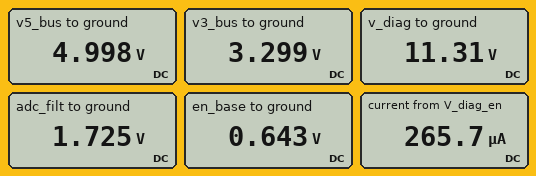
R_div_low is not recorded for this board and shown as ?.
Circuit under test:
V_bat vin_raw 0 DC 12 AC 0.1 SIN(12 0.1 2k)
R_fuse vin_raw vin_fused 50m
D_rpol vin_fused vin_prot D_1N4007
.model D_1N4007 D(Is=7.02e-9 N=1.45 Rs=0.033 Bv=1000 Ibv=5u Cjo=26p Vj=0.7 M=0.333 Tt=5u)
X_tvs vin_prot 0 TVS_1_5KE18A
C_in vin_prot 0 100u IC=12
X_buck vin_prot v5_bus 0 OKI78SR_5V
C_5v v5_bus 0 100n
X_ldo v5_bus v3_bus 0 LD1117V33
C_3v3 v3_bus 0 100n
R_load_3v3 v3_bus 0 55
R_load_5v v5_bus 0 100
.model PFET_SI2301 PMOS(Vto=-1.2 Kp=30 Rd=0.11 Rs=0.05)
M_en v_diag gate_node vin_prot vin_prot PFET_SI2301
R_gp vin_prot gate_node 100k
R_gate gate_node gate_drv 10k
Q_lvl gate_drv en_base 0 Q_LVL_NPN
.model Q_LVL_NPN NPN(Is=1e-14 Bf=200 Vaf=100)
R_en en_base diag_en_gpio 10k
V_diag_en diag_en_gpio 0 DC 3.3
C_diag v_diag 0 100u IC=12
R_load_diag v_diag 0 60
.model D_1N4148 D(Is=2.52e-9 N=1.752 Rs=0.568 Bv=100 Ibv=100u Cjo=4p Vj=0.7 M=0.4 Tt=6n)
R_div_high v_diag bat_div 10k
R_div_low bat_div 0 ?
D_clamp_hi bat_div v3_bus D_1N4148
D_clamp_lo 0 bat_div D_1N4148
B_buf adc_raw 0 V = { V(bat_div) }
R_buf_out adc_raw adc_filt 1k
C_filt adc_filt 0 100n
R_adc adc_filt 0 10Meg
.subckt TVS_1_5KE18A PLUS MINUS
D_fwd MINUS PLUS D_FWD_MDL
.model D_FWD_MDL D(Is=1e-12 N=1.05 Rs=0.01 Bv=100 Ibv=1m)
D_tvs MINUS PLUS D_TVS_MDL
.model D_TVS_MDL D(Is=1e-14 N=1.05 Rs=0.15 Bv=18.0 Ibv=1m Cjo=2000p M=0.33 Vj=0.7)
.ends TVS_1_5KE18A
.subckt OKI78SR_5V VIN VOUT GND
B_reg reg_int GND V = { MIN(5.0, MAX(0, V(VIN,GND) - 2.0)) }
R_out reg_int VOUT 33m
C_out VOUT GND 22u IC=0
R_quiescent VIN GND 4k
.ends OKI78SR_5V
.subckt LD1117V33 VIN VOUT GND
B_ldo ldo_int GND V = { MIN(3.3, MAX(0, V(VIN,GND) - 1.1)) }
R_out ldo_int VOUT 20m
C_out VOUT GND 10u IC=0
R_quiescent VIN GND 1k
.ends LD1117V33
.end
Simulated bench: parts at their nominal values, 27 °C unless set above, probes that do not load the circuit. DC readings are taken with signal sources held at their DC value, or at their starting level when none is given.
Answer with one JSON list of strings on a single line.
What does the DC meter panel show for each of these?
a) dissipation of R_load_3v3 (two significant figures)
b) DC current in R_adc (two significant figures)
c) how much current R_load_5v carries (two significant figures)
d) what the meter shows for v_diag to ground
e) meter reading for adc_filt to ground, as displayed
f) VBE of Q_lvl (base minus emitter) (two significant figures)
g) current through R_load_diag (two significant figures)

["200 mW", "170 nA", "50 mA", "11.31 V", "1.725 V", "640 mV", "190 mA"]
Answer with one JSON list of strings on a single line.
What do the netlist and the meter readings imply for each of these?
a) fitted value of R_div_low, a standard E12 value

["1.8 kΩ"]
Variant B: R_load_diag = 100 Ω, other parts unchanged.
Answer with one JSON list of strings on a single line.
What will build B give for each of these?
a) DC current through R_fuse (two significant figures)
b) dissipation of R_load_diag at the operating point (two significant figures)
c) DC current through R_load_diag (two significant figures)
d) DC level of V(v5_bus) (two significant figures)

["120 mA", "1.3 W", "110 mA", "5.0 V"]
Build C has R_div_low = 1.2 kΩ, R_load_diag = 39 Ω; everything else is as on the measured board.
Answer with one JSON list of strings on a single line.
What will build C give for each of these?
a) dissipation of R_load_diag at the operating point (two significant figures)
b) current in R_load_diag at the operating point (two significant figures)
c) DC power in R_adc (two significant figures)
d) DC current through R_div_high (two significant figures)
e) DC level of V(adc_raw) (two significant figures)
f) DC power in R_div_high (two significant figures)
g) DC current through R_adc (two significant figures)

["3.3 W", "290 mA", "150 nW", "1.0 mA", "1.2 V", "10 mW", "120 nA"]
